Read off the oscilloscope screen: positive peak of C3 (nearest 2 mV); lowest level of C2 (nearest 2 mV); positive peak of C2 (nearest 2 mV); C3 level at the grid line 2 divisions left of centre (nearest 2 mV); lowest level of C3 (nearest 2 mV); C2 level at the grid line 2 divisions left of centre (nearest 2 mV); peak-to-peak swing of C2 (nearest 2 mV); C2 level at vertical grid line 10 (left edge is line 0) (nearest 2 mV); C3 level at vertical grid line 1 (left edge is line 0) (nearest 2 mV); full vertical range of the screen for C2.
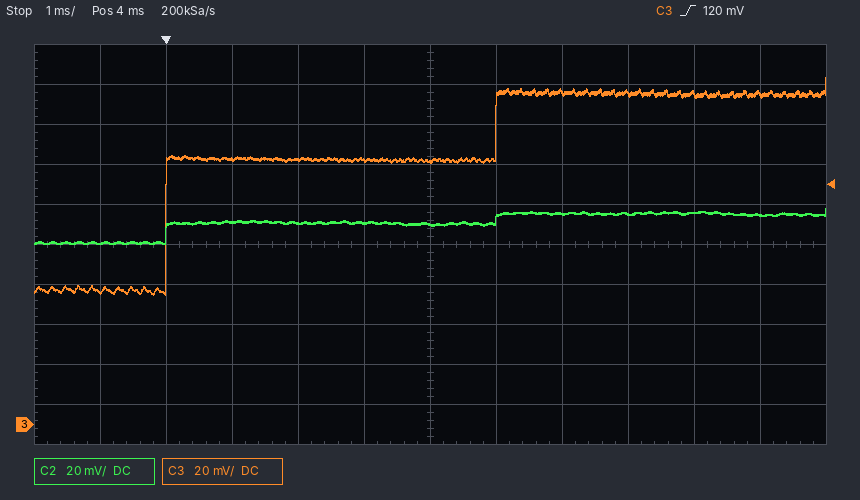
174 mV
90 mV
108 mV
132 mV
64 mV
100 mV
18 mV
106 mV
66 mV
200 mV
